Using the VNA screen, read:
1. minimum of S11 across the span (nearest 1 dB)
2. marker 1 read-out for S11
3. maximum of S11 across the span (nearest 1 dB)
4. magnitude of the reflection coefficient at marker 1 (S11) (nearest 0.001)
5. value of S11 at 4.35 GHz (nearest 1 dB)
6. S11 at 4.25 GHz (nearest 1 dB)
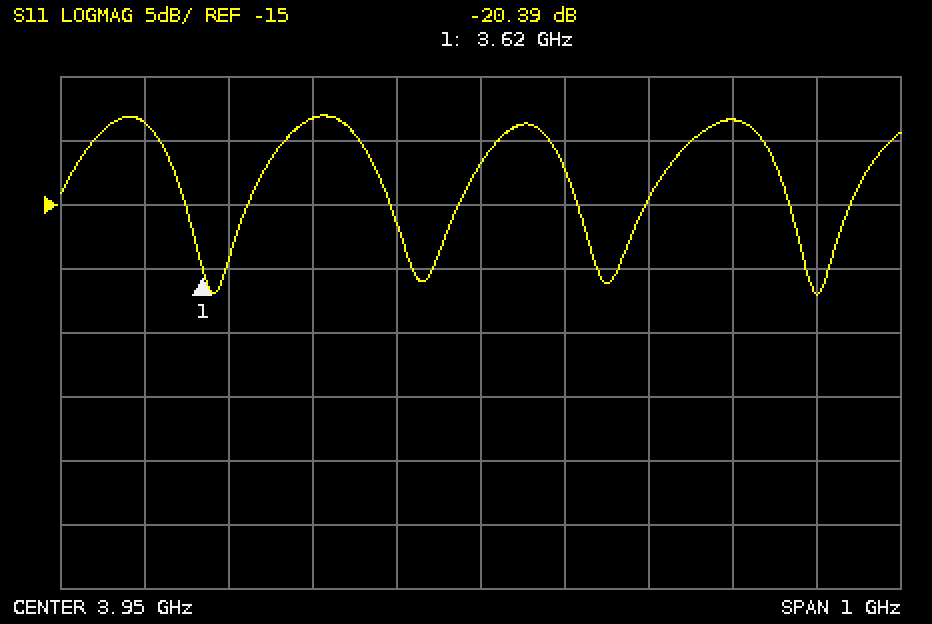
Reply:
-22 dB
-20.39 dB
-8 dB
0.096
-22 dB
-8 dB
